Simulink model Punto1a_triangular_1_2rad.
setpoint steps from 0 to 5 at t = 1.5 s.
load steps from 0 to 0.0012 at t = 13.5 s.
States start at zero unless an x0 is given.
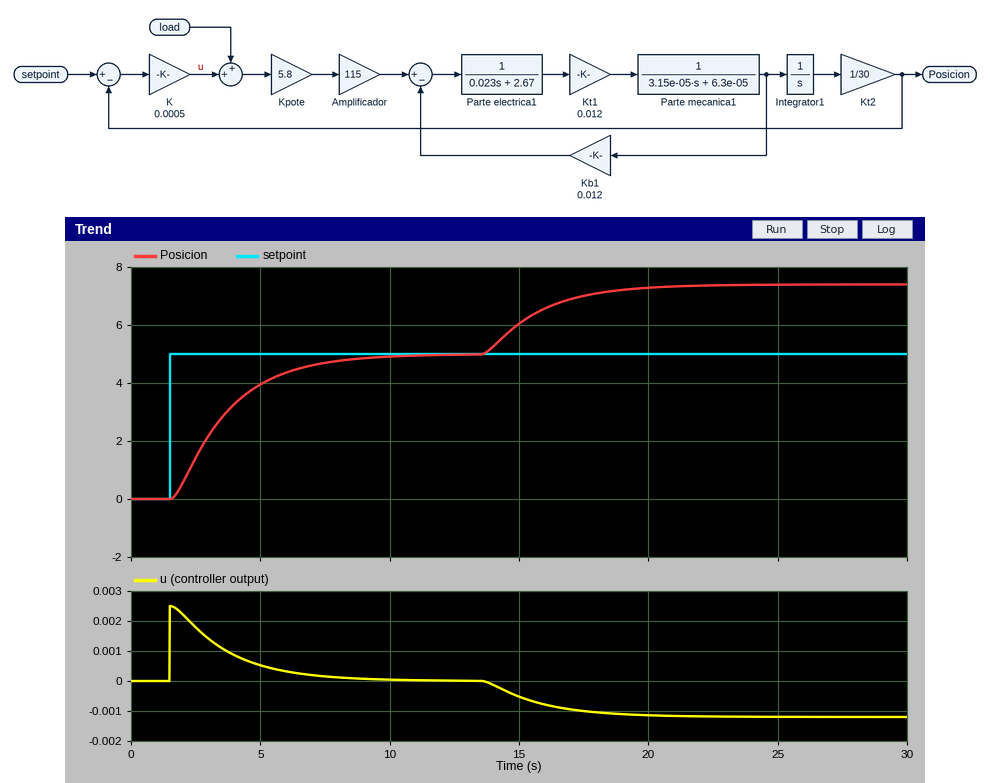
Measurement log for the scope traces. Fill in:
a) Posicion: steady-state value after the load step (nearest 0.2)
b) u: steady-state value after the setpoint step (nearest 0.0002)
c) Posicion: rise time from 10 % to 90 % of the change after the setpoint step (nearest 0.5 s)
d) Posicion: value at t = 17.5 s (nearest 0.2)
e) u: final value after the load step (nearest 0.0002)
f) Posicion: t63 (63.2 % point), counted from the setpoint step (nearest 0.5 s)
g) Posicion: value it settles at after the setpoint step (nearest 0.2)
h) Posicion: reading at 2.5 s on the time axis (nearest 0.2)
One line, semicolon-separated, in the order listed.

7.4; 0.0000; 4.5 s; 7.0; -0.0012; 2.5 s; 5.0; 1.4
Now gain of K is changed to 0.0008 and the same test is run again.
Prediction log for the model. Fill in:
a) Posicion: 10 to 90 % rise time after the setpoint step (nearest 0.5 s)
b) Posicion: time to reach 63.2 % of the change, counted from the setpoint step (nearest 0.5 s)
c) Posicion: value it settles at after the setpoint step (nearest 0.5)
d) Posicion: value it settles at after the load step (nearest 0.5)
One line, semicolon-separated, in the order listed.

2.5 s; 1.5 s; 5.0; 6.5
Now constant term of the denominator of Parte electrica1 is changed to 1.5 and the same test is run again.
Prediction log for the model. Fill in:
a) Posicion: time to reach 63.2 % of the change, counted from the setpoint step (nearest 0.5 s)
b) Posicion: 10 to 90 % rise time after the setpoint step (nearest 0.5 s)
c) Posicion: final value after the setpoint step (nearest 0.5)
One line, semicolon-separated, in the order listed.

2.0 s; 3.5 s; 5.0
